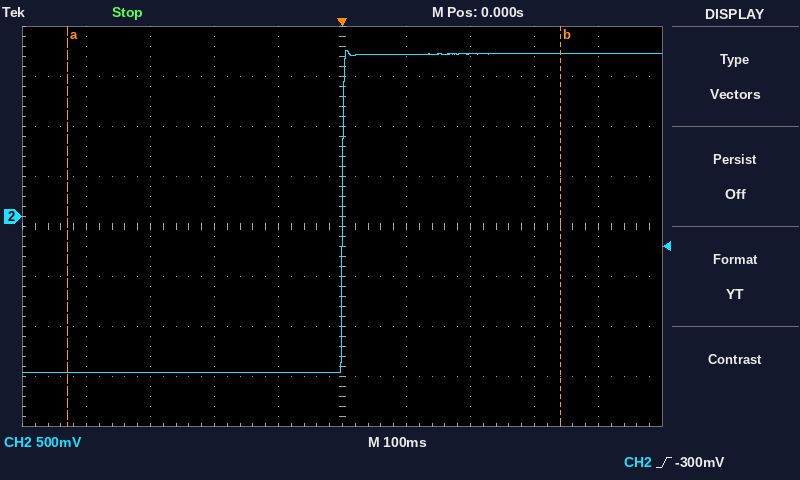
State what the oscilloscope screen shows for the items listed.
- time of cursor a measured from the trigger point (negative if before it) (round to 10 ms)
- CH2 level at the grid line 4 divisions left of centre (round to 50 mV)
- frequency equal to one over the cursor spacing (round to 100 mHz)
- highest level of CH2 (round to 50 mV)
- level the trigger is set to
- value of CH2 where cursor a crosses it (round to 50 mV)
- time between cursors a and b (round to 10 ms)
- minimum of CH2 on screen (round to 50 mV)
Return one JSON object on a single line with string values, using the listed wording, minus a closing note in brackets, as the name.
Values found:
{"time of cursor a measured from the trigger point (negative if before it)": "-430 ms", "CH2 level at the grid line 4 divisions left of centre": "-1.55 V", "frequency equal to one over the cursor spacing": "1.3 Hz", "highest level of CH2": "1.65 V", "level the trigger is set to": "-300 mV", "value of CH2 where cursor a crosses it": "-1.55 V", "time between cursors a and b": "770 ms", "minimum of CH2 on screen": "-1.55 V"}
